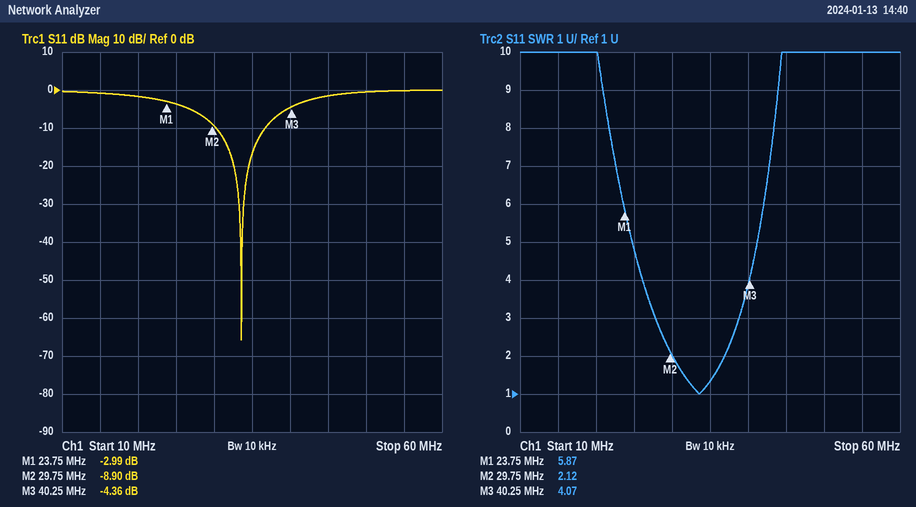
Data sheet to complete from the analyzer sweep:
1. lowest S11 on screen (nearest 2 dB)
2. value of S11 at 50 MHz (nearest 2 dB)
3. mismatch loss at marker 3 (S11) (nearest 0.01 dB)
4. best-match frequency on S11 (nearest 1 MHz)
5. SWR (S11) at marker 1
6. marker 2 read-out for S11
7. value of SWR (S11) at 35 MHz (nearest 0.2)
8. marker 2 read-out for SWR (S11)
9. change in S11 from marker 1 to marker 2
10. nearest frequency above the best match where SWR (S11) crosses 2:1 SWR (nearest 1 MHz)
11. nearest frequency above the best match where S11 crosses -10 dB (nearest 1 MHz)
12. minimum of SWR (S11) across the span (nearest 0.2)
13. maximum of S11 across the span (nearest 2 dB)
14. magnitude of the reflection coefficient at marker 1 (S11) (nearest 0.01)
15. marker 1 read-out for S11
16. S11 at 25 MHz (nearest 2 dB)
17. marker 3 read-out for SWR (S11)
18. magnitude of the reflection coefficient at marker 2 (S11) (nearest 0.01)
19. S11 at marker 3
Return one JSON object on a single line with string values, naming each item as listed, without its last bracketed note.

{"lowest S11 on screen": "-66 dB", "value of S11 at 50 MHz": "0 dB", "mismatch loss at marker 3 (S11)": "1.98 dB", "best-match frequency on S11": "34 MHz", "SWR (S11) at marker 1": "5.87", "marker 2 read-out for S11": "-8.90 dB", "value of SWR (S11) at 35 MHz": "1.4", "marker 2 read-out for SWR": "2.12", "change in S11 from marker 1 to marker 2": "-5.91 dB", "nearest frequency above the best match where SWR (S11) crosses 2:1 SWR": "37 MHz", "nearest frequency above the best match where S11 crosses -10 dB": "37 MHz", "minimum of SWR (S11) across the span": "1.0", "maximum of S11 across the span": "0 dB", "magnitude of the reflection coefficient at marker 1 (S11)": "0.71", "marker 1 read-out for S11": "-2.99 dB", "S11 at 25 MHz": "-4 dB", "marker 3 read-out for SWR": "4.07", "magnitude of the reflection coefficient at marker 2 (S11)": "0.36", "S11 at marker 3": "-4.36 dB"}
